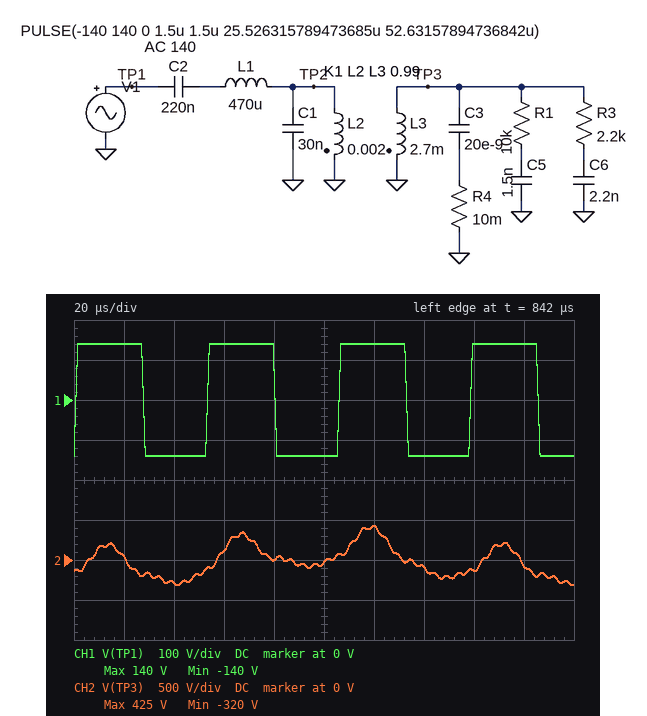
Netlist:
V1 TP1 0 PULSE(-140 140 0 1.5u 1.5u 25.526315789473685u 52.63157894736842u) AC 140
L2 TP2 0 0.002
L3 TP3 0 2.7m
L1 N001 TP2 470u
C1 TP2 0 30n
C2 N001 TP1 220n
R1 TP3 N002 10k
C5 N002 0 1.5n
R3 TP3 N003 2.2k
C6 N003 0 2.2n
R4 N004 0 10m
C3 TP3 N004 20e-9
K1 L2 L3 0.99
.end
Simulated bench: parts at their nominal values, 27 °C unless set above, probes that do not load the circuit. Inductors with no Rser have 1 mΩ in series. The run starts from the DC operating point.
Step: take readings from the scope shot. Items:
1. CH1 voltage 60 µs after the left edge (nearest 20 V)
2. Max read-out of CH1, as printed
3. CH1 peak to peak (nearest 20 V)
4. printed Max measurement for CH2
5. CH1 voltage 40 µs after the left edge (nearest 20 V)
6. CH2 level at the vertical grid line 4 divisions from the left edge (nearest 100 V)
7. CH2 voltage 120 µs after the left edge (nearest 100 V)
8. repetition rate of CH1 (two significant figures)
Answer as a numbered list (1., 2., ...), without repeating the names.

1. 140 V
2. 140 V
3. 280 V
4. 425 V
5. -140 V
6. 0 V
7. 400 V
8. 19 kHz
